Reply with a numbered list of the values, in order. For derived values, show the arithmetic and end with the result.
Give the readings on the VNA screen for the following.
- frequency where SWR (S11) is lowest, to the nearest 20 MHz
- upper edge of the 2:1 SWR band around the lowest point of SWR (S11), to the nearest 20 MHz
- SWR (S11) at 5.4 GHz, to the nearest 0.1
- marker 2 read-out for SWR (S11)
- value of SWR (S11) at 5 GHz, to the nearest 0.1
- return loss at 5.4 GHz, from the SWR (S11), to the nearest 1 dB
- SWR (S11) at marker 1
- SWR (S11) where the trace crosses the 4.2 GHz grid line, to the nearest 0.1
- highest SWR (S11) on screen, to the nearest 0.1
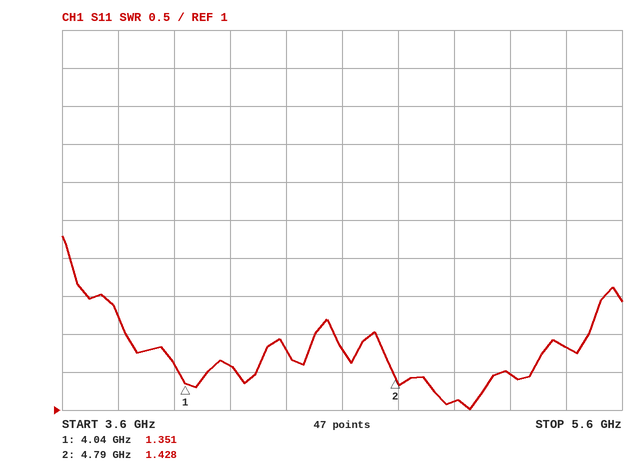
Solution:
1. 5.06 GHz
2. 5.48 GHz
3. 1.8
4. 1.428
5. 1.1
6. −20 log10((1.8 − 1)/(1.8 + 1)) ≈ 11 dB
7. 1.351
8. 1.6
9. 3.3
